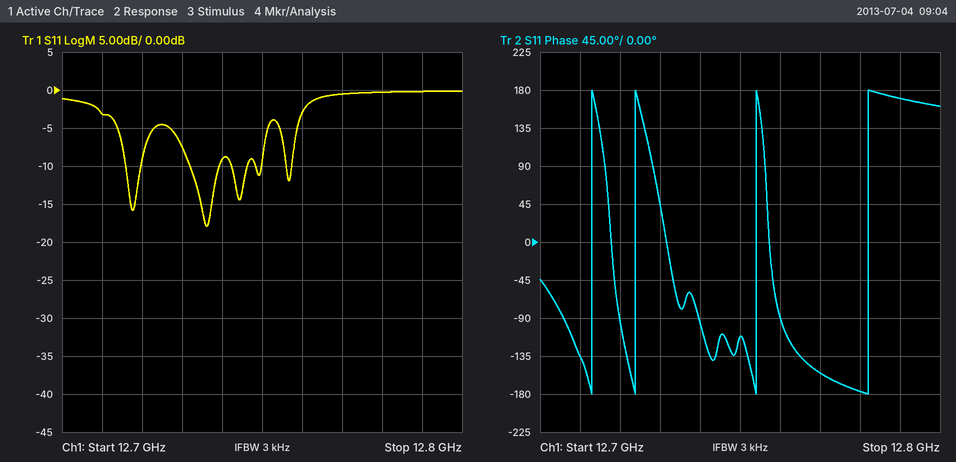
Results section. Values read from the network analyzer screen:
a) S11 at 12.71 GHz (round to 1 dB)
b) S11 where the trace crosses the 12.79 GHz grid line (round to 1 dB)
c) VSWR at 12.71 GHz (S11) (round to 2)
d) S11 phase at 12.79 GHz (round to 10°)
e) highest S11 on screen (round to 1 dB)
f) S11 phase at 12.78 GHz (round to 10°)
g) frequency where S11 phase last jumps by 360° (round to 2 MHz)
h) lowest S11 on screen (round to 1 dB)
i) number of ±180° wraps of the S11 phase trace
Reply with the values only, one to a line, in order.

-3 dB
0 dB
6
170°
0 dB
-180°
12.782 GHz
-18 dB
4
